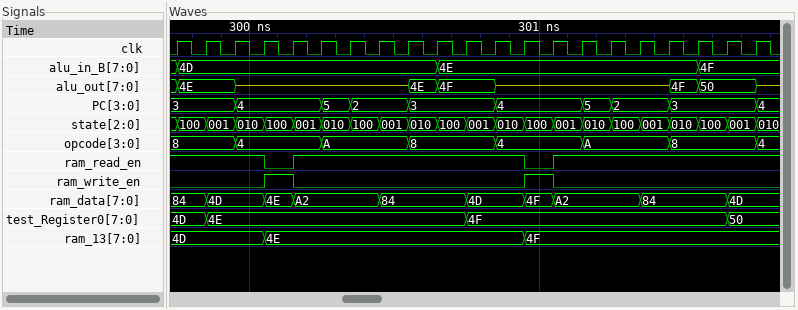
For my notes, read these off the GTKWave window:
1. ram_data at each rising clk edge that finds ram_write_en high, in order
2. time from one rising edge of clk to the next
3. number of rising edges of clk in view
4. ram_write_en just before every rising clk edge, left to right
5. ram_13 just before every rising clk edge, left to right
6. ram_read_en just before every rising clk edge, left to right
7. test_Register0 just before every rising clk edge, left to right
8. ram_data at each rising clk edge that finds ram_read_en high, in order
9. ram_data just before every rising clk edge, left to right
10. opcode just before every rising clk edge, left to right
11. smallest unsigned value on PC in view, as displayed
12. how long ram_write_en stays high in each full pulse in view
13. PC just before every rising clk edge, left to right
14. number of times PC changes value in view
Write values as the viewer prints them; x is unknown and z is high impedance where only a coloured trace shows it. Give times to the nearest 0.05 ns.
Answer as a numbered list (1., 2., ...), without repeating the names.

1. 4E, 4F
2. 0.1 ns
3. 21
4. 0 0 0 0 1 0 0 0 0 0 0 0 0 1 0 0 0 0 0 0 0
5. 4D, 4D, 4D, 4D, 4E, 4E, 4E, 4E, 4E, 4E, 4E, 4E, 4E, 4F, 4F, 4F, 4F, 4F, 4F, 4F, 4F
6. 1 1 1 1 0 1 1 1 1 1 1 1 1 0 1 1 1 1 1 1 1
7. 4D, 4D, 4E, 4E, 4E, 4E, 4E, 4E, 4E, 4E, 4E, 4F, 4F, 4F, 4F, 4F, 4F, 4F, 4F, 4F, 50
8. 84, 84, 4D, 4D, A2, A2, A2, 84, 84, 84, 4D, 4D, A2, A2, A2, 84, 84, 84, 4D
9. 84, 84, 4D, 4D, 4E, A2, A2, A2, 84, 84, 84, 4D, 4D, 4F, A2, A2, A2, 84, 84, 84, 4D
10. 8, 8, 8, 4, 4, 4, A, A, A, 8, 8, 8, 4, 4, 4, A, A, A, 8, 8, 8
11. 2
12. 0.1 ns, 0.1 ns
13. 3, 3, 3, 4, 4, 4, 5, 2, 2, 3, 3, 3, 4, 4, 4, 5, 2, 2, 3, 3, 3
14. 9
